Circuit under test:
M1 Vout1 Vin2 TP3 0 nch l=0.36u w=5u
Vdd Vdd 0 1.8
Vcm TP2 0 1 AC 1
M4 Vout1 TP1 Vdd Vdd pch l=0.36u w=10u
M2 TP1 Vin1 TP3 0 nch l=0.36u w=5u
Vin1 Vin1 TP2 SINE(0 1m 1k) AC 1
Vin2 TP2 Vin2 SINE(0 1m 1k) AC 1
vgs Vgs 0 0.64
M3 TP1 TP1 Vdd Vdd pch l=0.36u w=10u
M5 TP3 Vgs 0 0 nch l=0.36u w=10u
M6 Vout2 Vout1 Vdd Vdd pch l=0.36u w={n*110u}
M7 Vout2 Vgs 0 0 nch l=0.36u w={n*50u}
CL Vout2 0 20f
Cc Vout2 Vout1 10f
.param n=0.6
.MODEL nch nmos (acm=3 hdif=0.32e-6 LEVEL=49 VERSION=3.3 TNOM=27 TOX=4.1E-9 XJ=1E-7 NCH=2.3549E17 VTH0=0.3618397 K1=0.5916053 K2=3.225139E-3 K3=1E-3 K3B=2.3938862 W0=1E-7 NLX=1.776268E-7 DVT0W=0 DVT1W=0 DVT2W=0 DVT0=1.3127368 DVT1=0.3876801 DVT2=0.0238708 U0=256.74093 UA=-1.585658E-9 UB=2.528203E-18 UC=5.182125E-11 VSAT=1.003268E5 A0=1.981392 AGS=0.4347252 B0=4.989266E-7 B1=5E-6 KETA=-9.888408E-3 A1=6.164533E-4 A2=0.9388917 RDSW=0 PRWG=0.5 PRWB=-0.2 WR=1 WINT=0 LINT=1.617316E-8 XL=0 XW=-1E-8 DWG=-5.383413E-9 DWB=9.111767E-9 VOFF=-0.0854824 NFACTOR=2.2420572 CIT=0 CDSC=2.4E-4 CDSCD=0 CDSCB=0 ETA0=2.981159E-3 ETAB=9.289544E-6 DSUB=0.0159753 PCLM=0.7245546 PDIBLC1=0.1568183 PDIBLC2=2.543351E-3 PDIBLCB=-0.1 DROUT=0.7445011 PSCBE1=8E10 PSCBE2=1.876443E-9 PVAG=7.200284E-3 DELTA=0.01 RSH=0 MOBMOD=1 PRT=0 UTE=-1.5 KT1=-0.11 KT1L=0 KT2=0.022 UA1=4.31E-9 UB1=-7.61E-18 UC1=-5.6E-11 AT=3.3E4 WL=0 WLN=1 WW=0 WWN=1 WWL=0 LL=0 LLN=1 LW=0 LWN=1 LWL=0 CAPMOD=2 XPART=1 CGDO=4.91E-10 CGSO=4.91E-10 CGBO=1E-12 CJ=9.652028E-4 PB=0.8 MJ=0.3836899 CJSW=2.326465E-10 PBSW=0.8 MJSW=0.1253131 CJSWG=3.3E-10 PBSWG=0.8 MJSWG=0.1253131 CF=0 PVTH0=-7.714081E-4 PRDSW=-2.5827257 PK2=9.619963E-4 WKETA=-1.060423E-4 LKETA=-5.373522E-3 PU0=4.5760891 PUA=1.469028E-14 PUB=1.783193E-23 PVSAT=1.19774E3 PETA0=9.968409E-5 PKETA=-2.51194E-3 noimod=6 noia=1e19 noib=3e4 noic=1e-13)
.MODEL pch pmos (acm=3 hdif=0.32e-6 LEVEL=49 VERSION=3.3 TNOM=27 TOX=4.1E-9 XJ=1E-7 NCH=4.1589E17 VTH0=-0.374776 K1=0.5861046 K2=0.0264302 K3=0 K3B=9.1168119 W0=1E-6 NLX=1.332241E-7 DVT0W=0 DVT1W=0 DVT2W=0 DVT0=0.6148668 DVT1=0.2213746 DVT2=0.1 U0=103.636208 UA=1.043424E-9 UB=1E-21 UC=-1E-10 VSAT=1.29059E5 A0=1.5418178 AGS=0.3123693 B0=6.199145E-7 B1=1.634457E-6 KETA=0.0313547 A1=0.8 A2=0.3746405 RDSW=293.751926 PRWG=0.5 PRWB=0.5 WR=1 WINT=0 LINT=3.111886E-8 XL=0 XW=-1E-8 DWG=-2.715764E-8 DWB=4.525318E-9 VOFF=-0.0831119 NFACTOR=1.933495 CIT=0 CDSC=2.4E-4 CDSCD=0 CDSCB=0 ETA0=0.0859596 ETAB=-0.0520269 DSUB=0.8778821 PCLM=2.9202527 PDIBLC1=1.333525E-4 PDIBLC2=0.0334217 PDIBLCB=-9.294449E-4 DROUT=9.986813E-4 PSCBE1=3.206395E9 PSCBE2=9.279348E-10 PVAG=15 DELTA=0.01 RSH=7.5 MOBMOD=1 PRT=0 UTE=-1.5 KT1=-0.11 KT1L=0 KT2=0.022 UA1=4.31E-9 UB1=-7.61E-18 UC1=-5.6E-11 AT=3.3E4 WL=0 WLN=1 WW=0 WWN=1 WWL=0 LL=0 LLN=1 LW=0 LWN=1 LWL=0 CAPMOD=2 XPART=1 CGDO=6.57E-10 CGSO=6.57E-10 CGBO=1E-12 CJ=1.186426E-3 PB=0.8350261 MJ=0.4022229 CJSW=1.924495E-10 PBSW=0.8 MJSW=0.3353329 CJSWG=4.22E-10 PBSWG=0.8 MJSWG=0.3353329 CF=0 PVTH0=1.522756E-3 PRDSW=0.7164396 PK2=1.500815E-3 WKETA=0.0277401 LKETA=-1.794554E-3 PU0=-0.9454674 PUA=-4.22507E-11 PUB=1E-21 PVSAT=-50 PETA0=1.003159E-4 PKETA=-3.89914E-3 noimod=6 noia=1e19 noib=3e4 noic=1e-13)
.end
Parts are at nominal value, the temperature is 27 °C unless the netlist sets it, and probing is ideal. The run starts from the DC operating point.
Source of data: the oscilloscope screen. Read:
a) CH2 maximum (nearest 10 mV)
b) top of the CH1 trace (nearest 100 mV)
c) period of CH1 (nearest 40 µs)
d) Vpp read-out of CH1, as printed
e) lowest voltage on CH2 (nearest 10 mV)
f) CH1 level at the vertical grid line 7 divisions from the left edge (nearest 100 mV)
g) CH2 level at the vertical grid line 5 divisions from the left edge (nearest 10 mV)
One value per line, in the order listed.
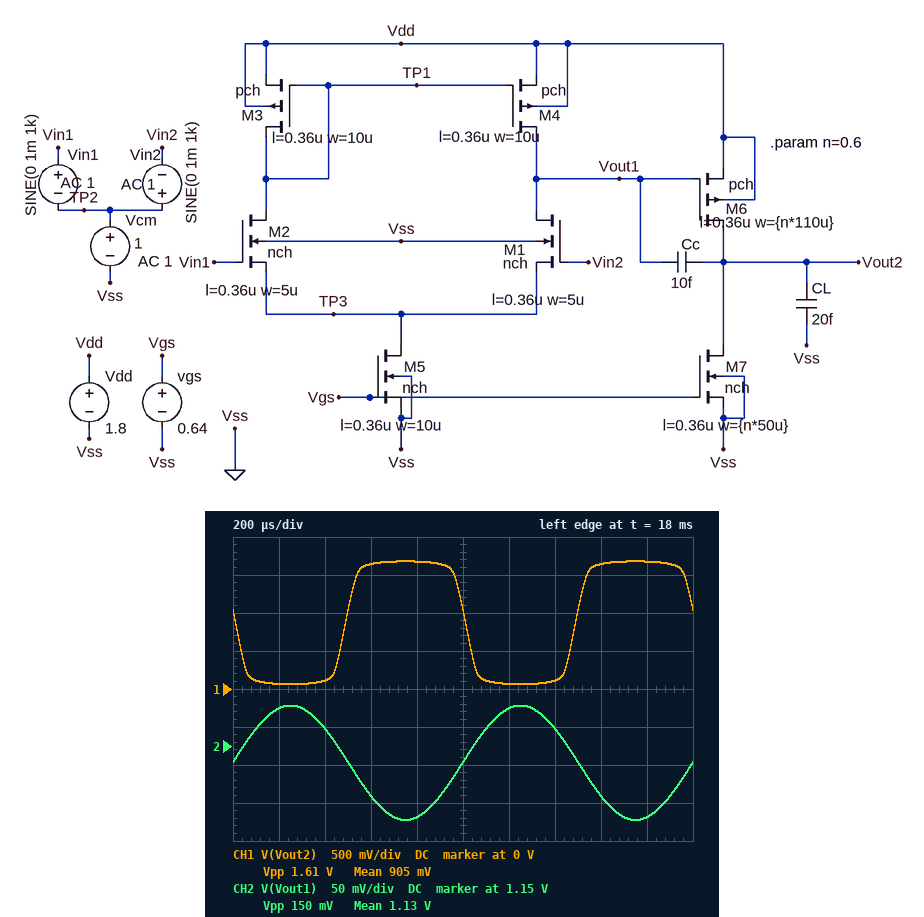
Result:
1.20 V
1.7 V
1.00 ms
1.61 V
1.05 V
100 mV
1.13 V
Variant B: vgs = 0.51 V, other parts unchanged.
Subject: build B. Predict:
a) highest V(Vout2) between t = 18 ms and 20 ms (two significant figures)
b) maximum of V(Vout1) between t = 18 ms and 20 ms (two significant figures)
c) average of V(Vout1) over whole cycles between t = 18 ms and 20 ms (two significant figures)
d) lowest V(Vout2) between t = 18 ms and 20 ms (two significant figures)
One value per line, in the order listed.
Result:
1.8 V
1.4 V
1.3 V
13 mV
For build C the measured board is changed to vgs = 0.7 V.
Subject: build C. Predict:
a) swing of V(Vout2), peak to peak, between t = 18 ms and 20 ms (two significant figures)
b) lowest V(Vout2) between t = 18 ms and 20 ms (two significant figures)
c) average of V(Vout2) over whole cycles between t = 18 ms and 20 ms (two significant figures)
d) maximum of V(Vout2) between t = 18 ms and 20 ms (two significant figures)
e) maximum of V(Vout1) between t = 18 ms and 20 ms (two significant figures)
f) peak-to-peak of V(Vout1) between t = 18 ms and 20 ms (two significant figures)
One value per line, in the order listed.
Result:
1.5 V
110 mV
890 mV
1.6 V
1.1 V
140 mV
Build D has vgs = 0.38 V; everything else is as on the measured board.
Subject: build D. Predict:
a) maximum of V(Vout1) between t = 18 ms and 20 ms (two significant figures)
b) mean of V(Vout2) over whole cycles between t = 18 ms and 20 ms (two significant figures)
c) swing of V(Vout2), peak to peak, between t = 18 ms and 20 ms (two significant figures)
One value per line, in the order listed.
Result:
1.5 V
940 mV
1.8 V
